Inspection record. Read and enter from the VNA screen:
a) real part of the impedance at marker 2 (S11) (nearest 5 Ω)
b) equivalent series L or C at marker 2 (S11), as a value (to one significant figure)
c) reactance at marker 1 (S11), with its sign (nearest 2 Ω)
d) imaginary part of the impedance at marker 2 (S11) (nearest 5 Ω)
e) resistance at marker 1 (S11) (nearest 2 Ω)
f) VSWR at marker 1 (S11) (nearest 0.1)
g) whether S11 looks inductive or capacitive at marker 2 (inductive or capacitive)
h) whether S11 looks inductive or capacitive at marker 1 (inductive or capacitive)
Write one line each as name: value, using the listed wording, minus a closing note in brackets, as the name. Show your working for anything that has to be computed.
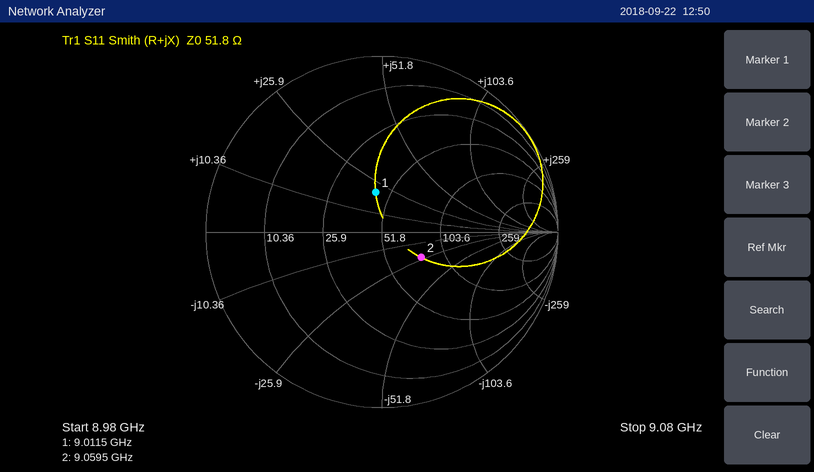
real part of the impedance at marker 2 (S11): 75 Ω
equivalent series L or C at marker 2 (S11), as a value: C = 1/(2π × 9.0595 GHz × 25 Ω) ≈ 703 fF, so 700 fF to one significant figure
reactance at marker 1 (S11), with its sign: +20 Ω
imaginary part of the impedance at marker 2 (S11): -25 Ω
resistance at marker 1 (S11): 44 Ω
VSWR at marker 1 (S11): 1.6
whether S11 looks inductive or capacitive at marker 2: capacitive
whether S11 looks inductive or capacitive at marker 1: inductive
